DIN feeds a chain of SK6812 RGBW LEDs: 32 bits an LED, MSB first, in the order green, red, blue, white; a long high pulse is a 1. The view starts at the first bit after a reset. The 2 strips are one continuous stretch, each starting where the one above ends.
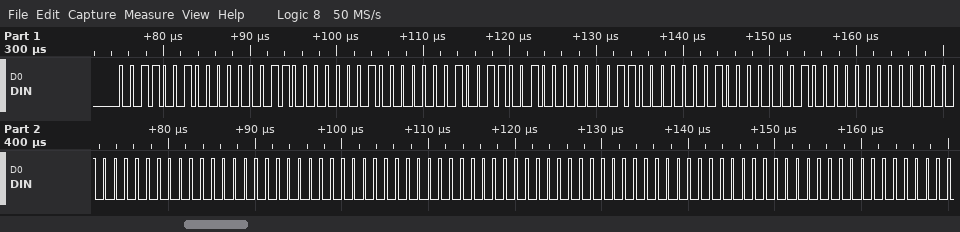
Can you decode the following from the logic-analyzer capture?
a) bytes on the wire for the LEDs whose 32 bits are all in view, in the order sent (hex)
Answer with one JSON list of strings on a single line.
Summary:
["32 03 01 01 32 03 01 01 00 00 00 00 00 00 00 00"]
